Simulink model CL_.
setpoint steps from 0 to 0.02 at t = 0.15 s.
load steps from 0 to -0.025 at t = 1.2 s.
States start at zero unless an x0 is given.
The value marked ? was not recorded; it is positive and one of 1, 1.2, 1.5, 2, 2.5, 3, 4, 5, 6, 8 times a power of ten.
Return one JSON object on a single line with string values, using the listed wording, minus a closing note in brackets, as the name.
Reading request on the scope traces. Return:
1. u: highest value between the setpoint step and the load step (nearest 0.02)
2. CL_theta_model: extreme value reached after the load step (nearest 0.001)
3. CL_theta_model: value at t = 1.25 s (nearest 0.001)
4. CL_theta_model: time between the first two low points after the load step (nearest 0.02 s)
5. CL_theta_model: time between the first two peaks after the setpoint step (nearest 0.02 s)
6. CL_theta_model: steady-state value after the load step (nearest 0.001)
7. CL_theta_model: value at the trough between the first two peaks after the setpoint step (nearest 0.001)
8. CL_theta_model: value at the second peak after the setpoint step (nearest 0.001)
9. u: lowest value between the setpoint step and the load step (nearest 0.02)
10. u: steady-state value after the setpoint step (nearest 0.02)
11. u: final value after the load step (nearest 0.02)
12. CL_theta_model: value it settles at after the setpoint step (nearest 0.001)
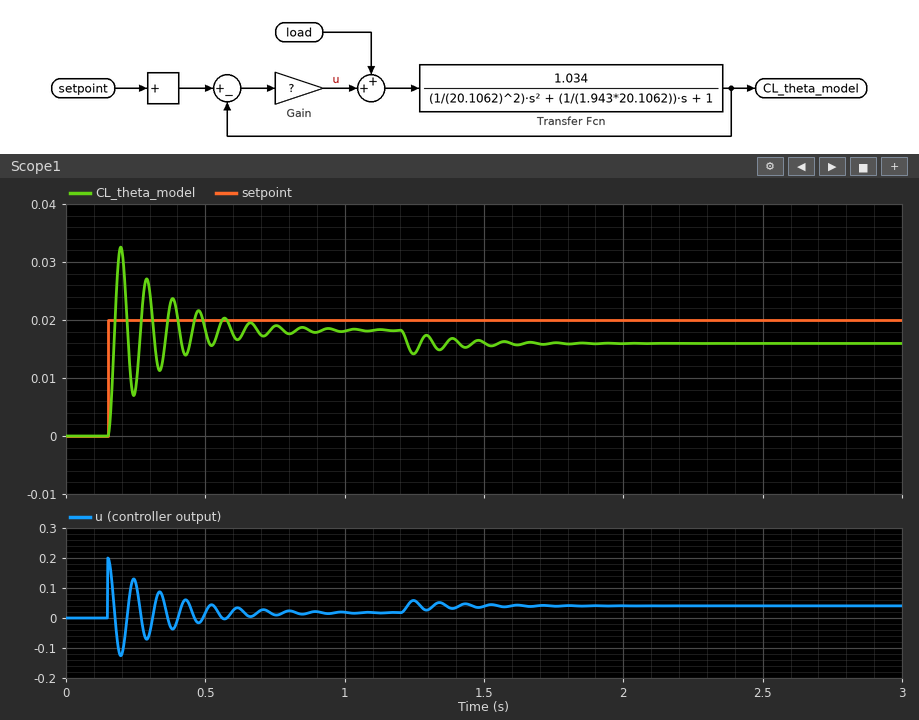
{"u: highest value between the setpoint step and the load step": "0.20", "CL_theta_model: extreme value reached after the load step": "0.014", "CL_theta_model: value at t = 1.25 s": "0.014", "CL_theta_model: time between the first two low points after the load step": "0.10 s", "CL_theta_model: time between the first two peaks after the setpoint step": "0.10 s", "CL_theta_model: steady-state value after the load step": "0.016", "CL_theta_model: value at the trough between the first two peaks after the setpoint step": "0.007", "CL_theta_model: value at the second peak after the setpoint step": "0.027", "u: lowest value between the setpoint step and the load step": "-0.12", "u: steady-state value after the setpoint step": "0.02", "u: final value after the load step": "0.04", "CL_theta_model: value it settles at after the setpoint step": "0.018"}
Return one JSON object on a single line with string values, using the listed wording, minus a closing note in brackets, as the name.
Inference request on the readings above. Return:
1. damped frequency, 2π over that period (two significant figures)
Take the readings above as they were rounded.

{"damped frequency, 2π over that period": "63 rad/s"}
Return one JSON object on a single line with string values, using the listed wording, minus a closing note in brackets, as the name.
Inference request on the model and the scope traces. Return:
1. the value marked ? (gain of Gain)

{"the value marked ?": "10"}
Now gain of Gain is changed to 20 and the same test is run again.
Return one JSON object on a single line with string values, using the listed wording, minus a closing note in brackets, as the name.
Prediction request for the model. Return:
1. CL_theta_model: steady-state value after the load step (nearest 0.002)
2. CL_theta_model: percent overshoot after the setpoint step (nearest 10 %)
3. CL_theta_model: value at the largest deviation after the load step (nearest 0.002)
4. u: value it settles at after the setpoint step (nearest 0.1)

{"CL_theta_model: steady-state value after the load step": "0.018", "CL_theta_model: percent overshoot after the setpoint step": "80 %", "CL_theta_model: value at the largest deviation after the load step": "0.016", "u: value it settles at after the setpoint step": "0.0"}
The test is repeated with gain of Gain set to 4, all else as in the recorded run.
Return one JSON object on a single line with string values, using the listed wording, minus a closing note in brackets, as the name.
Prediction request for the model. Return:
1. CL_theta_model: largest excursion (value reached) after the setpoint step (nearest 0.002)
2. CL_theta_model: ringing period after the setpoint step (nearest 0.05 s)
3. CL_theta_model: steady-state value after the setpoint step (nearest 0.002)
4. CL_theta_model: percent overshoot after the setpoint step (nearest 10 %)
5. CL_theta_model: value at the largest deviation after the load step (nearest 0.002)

{"CL_theta_model: largest excursion (value reached) after the setpoint step": "0.028", "CL_theta_model: ringing period after the setpoint step": "0.15 s", "CL_theta_model: steady-state value after the setpoint step": "0.016", "CL_theta_model: percent overshoot after the setpoint step": "70 %", "CL_theta_model: value at the largest deviation after the load step": "0.008"}
